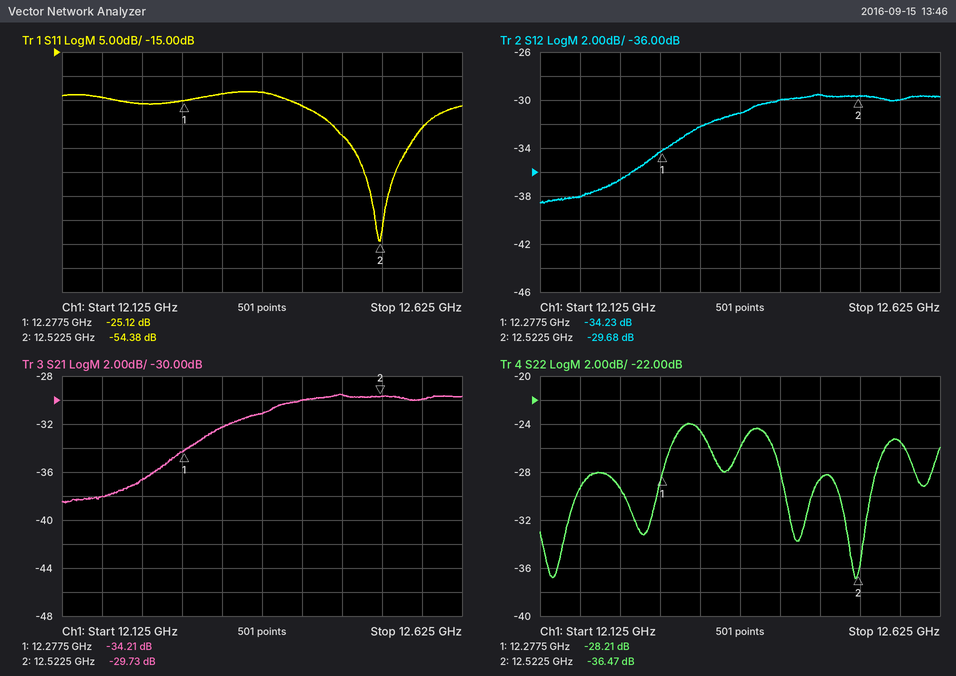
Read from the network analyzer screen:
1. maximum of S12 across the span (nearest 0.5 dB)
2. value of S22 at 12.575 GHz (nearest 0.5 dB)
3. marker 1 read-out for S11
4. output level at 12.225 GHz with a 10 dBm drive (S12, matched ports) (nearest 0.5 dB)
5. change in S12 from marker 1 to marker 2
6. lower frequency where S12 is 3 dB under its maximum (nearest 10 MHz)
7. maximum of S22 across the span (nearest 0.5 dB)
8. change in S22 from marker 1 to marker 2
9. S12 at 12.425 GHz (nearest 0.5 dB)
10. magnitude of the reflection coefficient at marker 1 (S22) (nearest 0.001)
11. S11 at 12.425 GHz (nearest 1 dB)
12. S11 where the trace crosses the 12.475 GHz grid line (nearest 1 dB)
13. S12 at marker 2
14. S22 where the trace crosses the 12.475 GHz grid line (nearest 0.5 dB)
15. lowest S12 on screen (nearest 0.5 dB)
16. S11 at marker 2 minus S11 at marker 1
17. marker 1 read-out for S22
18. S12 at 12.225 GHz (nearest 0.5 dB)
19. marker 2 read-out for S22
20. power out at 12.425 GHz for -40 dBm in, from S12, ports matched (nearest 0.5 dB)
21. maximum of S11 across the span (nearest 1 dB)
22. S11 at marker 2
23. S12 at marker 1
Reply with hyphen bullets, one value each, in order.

- -29.5 dB
- -25.5 dB
- -25.12 dB
- -26.5 dBm
- 4.55 dB
- 12.32 GHz
- -24.0 dB
- -8.26 dB
- -30.0 dB
- 0.039
- -26 dB
- -32 dB
- -29.68 dB
- -28.5 dB
- -38.5 dB
- -29.26 dB
- -28.21 dB
- -36.5 dB
- -36.47 dB
- -70.0 dBm
- -23 dB
- -54.38 dB
- -34.23 dB
